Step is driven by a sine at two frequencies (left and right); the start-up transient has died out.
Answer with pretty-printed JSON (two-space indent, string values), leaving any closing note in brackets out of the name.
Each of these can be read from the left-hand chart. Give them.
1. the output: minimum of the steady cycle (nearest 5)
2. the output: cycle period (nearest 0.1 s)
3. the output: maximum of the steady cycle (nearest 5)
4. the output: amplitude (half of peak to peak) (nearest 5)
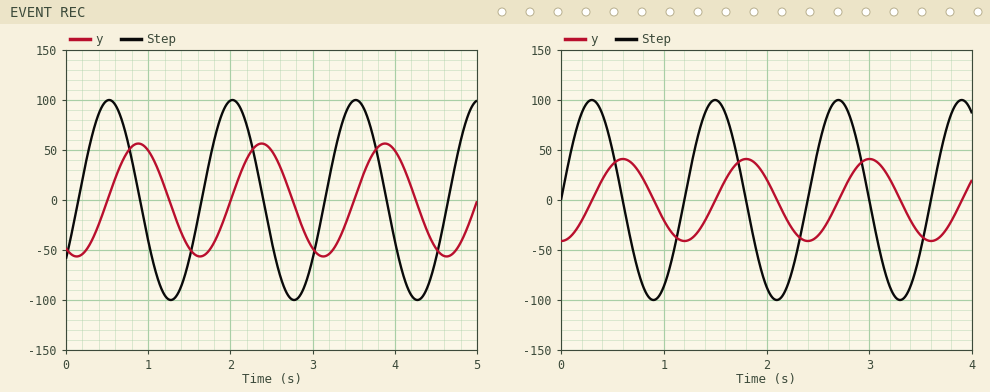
{
  "the output: minimum of the steady cycle": "-55",
  "the output: cycle period": "1.5 s",
  "the output: maximum of the steady cycle": "55",
  "the output: amplitude (half of peak to peak)": "55"
}
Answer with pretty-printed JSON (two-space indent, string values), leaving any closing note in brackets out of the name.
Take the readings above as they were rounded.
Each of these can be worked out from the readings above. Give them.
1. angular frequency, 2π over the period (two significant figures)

{
  "angular frequency, 2π over the period": "4.2 rad/s"
}
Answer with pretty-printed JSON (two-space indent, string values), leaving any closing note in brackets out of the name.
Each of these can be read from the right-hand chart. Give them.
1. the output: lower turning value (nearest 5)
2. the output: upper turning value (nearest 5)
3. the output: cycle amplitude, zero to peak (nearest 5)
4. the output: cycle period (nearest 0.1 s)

{
  "the output: lower turning value": "-40",
  "the output: upper turning value": "40",
  "the output: cycle amplitude, zero to peak": "40",
  "the output: cycle period": "1.2 s"
}
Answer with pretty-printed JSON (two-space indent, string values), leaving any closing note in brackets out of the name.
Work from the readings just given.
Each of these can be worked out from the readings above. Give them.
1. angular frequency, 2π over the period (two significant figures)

{
  "angular frequency, 2π over the period": "5.2 rad/s"
}
